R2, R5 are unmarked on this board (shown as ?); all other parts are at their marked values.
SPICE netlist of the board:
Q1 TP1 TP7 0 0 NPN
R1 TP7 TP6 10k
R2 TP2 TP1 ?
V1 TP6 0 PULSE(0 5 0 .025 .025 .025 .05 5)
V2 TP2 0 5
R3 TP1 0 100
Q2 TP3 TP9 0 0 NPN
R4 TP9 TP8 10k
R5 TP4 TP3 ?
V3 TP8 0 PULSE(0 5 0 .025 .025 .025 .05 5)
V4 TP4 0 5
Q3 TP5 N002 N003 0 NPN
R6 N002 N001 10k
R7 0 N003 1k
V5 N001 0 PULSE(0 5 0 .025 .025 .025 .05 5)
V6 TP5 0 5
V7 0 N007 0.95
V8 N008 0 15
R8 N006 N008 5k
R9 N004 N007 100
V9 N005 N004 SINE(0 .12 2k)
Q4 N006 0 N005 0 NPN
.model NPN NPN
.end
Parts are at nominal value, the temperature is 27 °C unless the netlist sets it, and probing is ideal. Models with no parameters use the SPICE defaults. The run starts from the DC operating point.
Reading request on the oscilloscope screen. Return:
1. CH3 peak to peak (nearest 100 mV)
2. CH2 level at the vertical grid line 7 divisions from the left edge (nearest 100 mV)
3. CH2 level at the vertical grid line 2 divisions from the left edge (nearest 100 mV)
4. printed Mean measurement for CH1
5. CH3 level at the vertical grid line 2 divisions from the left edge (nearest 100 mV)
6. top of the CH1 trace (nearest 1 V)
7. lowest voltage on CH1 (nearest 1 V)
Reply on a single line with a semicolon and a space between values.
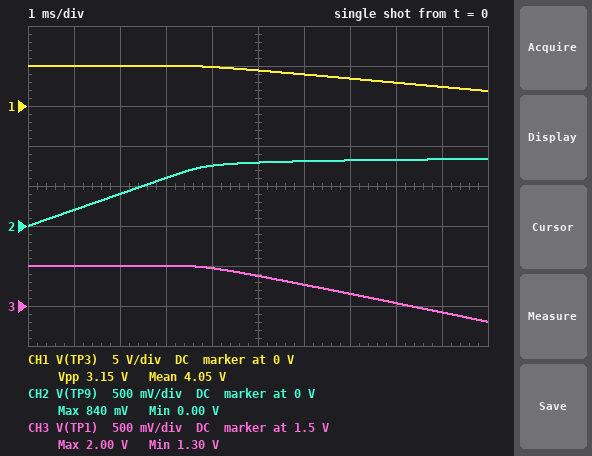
700 mV; 800 mV; 400 mV; 4.05 V; 2.0 V; 5 V; 2 V
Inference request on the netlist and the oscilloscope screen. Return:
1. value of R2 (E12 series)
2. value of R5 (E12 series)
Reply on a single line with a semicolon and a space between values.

150 Ω; 270 Ω
